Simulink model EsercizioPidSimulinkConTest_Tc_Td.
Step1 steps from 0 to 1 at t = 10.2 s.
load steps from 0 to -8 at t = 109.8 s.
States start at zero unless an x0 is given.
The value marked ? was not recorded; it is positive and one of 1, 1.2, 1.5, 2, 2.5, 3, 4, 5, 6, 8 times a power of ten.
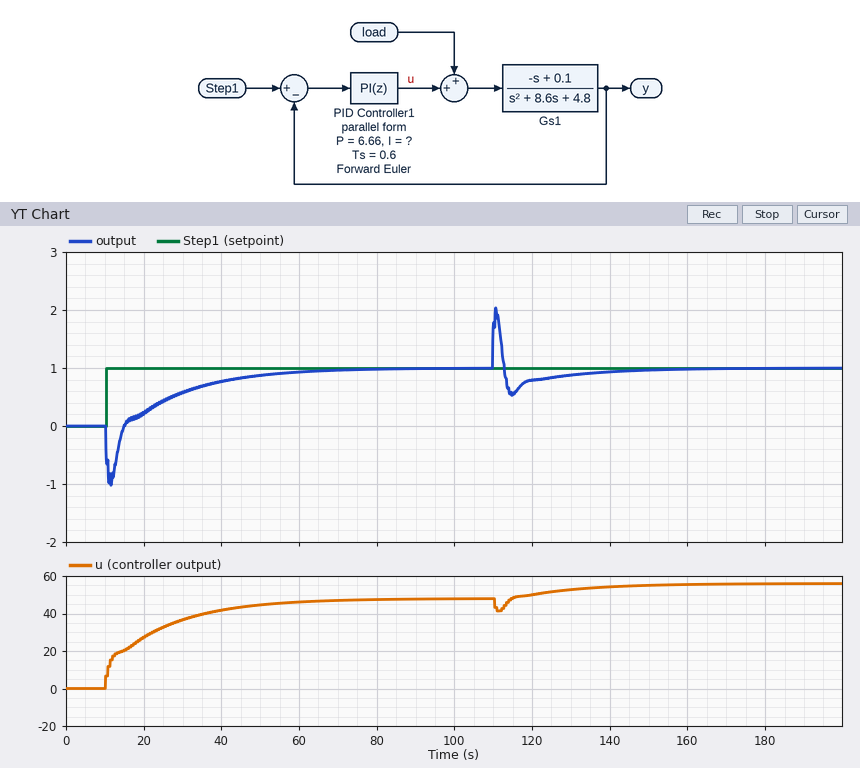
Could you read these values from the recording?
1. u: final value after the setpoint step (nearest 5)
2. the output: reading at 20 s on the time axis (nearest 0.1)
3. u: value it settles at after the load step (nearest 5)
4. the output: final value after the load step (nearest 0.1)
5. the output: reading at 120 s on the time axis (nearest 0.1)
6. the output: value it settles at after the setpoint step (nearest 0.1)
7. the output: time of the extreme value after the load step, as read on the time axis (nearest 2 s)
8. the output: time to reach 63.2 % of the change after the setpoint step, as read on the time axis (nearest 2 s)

50
0.2
55
1.0
0.8
1.0
110 s
32 s
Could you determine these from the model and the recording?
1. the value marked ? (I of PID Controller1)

2
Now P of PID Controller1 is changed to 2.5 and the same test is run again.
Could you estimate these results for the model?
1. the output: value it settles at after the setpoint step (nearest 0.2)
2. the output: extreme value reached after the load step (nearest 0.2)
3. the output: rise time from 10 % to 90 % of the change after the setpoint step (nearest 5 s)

1.0
1.8
30 s
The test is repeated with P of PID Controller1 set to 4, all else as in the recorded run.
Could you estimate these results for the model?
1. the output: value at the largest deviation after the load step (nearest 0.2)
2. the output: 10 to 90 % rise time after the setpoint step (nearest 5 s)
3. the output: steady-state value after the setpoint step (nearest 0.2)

1.8
30 s
1.0
